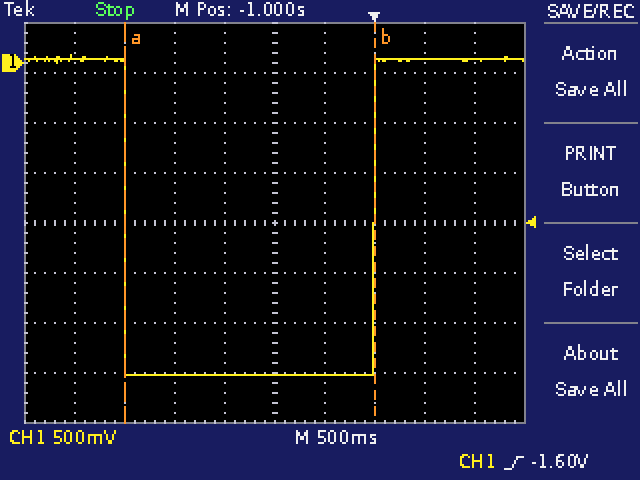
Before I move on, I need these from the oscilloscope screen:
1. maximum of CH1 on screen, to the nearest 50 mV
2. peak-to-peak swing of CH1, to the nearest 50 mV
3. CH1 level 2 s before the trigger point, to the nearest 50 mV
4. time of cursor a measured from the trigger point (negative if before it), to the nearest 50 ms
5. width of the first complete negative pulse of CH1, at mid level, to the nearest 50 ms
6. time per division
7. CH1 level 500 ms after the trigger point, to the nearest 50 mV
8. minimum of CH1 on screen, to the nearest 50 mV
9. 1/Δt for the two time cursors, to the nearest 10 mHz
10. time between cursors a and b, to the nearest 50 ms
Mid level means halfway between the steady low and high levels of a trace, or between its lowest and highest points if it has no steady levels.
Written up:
100 mV
3.20 V
-3.10 V
-2.50 s
2.50 s
500 ms
50 mV
-3.10 V
400 mHz
2.50 s
